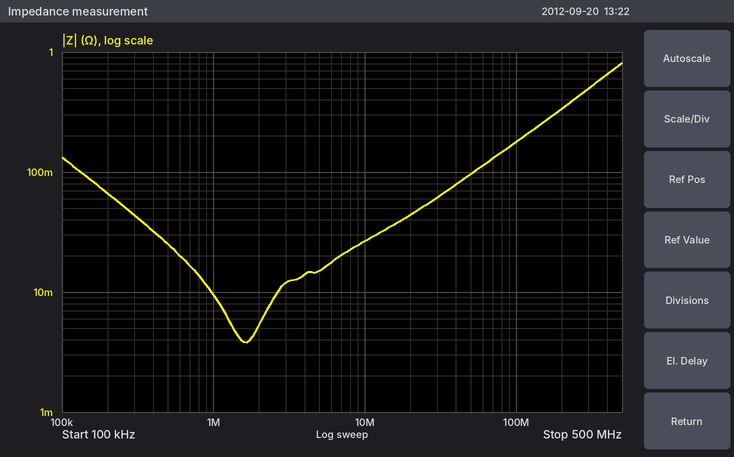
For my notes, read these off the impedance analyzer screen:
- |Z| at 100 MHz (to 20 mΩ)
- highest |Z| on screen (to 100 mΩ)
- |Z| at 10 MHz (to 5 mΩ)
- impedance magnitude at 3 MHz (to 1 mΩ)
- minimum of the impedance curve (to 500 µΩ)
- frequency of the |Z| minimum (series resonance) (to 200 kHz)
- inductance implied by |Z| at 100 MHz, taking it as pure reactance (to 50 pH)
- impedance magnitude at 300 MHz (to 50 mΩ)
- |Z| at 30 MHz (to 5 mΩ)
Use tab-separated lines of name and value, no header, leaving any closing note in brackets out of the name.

|Z| at 100 MHz	180 mΩ
highest |Z| on screen	800 mΩ
|Z| at 10 MHz	25 mΩ
impedance magnitude at 3 MHz	12 mΩ
minimum of the impedance curve	4.0 mΩ
frequency of the |Z| minimum (series resonance)	1.6 MHz
inductance implied by |Z| at 100 MHz, taking it as pure reactance	300 pH
impedance magnitude at 300 MHz	500 mΩ
|Z| at 30 MHz	60 mΩ
